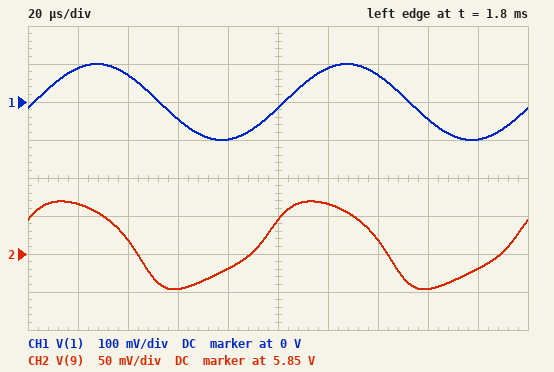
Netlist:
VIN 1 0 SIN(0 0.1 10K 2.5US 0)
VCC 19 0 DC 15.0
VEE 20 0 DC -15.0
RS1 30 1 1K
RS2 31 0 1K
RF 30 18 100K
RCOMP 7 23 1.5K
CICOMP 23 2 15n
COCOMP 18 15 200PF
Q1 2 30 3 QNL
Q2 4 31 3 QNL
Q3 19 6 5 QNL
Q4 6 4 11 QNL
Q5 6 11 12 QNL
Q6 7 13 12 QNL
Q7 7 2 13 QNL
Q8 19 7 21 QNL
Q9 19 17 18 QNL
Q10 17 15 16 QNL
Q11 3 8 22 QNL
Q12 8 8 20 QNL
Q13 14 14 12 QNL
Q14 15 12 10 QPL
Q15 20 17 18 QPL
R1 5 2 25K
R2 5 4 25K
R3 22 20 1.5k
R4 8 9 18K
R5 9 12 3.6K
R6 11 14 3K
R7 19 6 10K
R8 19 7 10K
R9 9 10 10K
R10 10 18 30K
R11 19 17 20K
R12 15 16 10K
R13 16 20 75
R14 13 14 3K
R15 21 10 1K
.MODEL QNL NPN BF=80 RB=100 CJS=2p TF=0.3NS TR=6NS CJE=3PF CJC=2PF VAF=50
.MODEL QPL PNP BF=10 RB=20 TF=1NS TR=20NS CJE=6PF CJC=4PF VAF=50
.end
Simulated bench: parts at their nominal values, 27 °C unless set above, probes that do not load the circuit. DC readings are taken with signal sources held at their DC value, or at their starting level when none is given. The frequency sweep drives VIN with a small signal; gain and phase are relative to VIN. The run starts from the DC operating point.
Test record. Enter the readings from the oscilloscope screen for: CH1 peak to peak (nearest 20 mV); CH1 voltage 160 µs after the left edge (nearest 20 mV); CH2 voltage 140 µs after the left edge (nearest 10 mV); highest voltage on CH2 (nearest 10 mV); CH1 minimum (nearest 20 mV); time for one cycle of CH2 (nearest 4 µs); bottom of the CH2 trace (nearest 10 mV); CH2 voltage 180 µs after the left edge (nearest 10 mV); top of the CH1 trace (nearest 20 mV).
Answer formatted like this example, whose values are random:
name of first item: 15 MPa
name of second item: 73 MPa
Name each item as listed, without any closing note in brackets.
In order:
CH1 peak to peak: 200 mV
CH1 voltage 160 µs after the left edge: -40 mV
CH2 voltage 140 µs after the left edge: 5.87 V
highest voltage on CH2: 5.92 V
CH1 minimum: -100 mV
time for one cycle of CH2: 100 µs
bottom of the CH2 trace: 5.80 V
CH2 voltage 180 µs after the left edge: 5.83 V
top of the CH1 trace: 100 mV
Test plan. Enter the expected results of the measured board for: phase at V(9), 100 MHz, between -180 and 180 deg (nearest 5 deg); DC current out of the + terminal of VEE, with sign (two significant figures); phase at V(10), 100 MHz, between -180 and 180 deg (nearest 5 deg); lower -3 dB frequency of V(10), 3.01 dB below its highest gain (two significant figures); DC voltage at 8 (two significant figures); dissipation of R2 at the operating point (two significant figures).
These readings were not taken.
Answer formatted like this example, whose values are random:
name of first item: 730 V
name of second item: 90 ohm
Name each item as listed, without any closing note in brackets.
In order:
phase at V(9), 100 MHz, between -180 and 180 deg: -30 deg
DC current out of the + terminal of VEE, with sign: -2.4 mA
phase at V(10), 100 MHz, between -180 and 180 deg: -30 deg
lower -3 dB frequency of V(10), 3.01 dB below its highest gain: 750 kHz
DC voltage at 8: -14 V
dissipation of R2 at the operating point: 20 µW
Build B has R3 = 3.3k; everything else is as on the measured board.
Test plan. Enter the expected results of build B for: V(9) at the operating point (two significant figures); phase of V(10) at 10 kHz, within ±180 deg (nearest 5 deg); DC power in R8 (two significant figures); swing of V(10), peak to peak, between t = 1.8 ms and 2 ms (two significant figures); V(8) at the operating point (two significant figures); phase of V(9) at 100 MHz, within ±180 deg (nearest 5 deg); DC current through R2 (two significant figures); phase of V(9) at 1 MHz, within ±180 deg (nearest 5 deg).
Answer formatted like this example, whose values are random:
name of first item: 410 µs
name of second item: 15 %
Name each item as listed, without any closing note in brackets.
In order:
V(9) at the operating point: 6.0 V
phase of V(10) at 10 kHz, within ±180 deg: 40 deg
DC power in R8: 1.6 mW
swing of V(10), peak to peak, between t = 1.8 ms and 2 ms: 95 mV
V(8) at the operating point: -14 V
phase of V(9) at 100 MHz, within ±180 deg: -45 deg
DC current through R2: 15 µA
phase of V(9) at 1 MHz, within ±180 deg: 5 deg
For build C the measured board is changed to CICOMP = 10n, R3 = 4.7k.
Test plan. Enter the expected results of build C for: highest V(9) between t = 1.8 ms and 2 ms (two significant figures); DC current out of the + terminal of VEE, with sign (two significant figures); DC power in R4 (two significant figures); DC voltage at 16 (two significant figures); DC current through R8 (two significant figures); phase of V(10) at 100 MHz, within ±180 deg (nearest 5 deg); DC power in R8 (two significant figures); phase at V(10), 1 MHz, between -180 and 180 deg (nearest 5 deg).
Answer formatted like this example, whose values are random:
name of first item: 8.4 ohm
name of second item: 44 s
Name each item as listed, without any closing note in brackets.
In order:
highest V(9) between t = 1.8 ms and 2 ms: 6.1 V
DC current out of the + terminal of VEE, with sign: -2.3 mA
DC power in R4: 23 mW
DC voltage at 16: -15 V
DC current through R8: 400 µA
phase of V(10) at 100 MHz, within ±180 deg: -45 deg
DC power in R8: 1.6 mW
phase at V(10), 1 MHz, between -180 and 180 deg: 0 deg
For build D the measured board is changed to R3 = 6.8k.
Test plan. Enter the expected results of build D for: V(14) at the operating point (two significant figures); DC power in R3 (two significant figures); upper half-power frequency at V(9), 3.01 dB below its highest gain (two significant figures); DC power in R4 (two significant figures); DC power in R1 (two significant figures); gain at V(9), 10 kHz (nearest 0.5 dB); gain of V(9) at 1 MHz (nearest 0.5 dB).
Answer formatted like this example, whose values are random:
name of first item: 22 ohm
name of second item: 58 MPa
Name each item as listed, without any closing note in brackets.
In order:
V(14) at the operating point: 9.5 V
DC power in R3: 2.0 µW
upper half-power frequency at V(9), 3.01 dB below its highest gain: 950 Hz
DC power in R4: 23 mW
DC power in R1: 1.9 µW
gain at V(9), 10 kHz: -8.5 dB
gain of V(9) at 1 MHz: -4.5 dB
